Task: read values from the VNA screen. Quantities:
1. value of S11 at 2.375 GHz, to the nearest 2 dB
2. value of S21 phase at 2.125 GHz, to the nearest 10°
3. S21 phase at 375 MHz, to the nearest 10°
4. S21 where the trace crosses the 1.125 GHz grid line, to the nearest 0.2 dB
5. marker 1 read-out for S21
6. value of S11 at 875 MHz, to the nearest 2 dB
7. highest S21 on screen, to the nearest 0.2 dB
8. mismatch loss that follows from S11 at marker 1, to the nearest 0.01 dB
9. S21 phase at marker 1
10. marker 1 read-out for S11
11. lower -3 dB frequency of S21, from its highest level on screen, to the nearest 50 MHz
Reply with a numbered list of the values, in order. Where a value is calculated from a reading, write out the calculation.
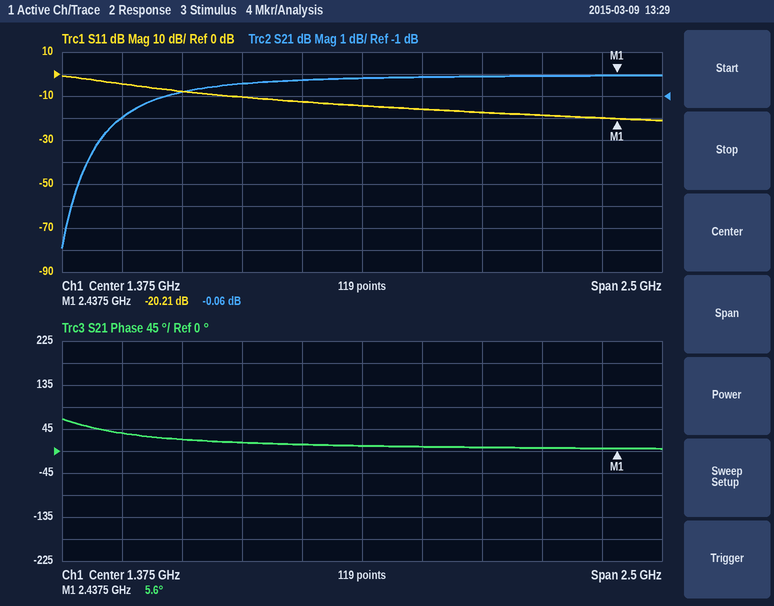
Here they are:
1. -20 dB
2. 10°
3. 40°
4. -0.2 dB
5. -0.06 dB
6. -10 dB
7. 0.0 dB
8. −10 log10(1 − 10^(-20.21/10)) ≈ 0.04 dB
9. 5.6°
10. -20.21 dB
11. 300 MHz
